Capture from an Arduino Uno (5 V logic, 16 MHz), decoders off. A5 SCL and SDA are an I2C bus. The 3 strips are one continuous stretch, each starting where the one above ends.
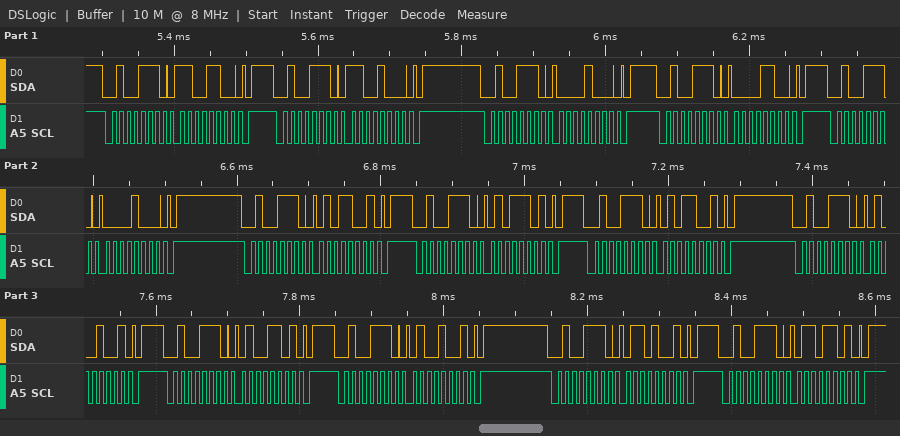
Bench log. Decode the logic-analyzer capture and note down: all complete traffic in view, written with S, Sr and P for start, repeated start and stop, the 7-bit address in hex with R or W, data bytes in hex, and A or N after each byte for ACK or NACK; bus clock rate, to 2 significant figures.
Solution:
S 27W A CC A P S 27W A C8 A P S 27W A 08 A P S 27W A 0C A P S 27W A 08 A P S 27W A 59 A P S 27W A 5D A P S 27W A 59 A P S 27W A 49 A P S 27W A 4D A P S 27W A 49 A P S 27W A 69 A P S 27W A 6D A P
100 kHz
